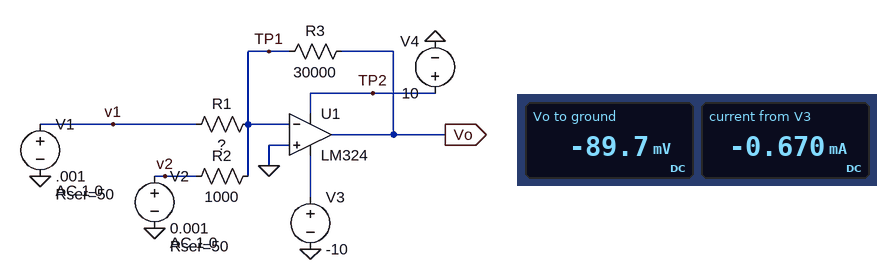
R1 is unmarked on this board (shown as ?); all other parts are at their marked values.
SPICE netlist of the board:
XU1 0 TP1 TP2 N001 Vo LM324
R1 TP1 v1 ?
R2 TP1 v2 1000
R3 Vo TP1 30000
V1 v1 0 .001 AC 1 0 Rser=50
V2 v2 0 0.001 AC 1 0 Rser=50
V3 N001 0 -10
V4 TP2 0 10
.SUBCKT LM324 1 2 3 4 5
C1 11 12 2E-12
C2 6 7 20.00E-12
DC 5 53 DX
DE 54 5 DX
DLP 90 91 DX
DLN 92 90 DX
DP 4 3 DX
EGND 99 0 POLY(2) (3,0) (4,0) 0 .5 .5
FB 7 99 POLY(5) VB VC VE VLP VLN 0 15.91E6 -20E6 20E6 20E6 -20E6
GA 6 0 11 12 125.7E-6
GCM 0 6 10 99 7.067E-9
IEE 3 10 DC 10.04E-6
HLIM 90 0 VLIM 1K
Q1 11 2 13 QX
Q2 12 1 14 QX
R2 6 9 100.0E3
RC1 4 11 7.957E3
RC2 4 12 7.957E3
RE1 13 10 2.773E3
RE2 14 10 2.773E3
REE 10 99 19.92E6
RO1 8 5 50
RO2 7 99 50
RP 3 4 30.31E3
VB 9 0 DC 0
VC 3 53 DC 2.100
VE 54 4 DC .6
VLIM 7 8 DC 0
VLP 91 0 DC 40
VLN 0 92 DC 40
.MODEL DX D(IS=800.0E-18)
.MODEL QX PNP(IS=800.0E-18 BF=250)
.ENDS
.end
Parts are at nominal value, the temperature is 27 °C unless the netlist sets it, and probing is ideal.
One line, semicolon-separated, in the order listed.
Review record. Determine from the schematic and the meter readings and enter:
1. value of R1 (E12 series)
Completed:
470 Ω
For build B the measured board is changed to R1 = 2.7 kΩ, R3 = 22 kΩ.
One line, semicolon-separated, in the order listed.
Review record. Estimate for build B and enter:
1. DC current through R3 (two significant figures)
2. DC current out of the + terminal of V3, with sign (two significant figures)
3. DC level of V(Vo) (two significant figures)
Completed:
1.4 µA; -670 µA; -30 mV
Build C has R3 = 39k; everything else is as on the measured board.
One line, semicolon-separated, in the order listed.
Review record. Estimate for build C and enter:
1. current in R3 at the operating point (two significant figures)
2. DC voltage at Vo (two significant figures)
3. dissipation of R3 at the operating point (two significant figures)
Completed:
3.0 µA; -120 mV; 350 nW
